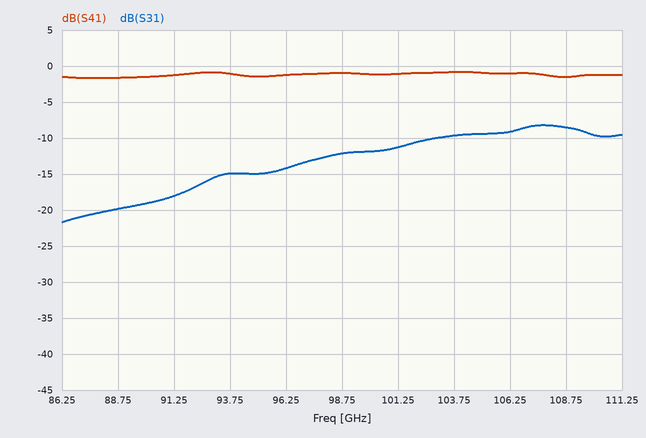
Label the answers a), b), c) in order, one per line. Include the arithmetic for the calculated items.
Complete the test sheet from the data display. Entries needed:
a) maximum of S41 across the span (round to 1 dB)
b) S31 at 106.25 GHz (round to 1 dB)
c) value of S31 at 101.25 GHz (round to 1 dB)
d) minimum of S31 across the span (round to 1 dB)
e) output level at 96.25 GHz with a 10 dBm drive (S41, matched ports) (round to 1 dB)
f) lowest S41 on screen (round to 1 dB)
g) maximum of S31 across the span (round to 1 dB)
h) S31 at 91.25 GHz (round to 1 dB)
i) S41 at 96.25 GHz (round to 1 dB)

a) -1 dB
b) -9 dB
c) -11 dB
d) -22 dB
e) 10 dBm + (-1 dB) = 9 dBm
f) -2 dB
g) -8 dB
h) -18 dB
i) -1 dB
